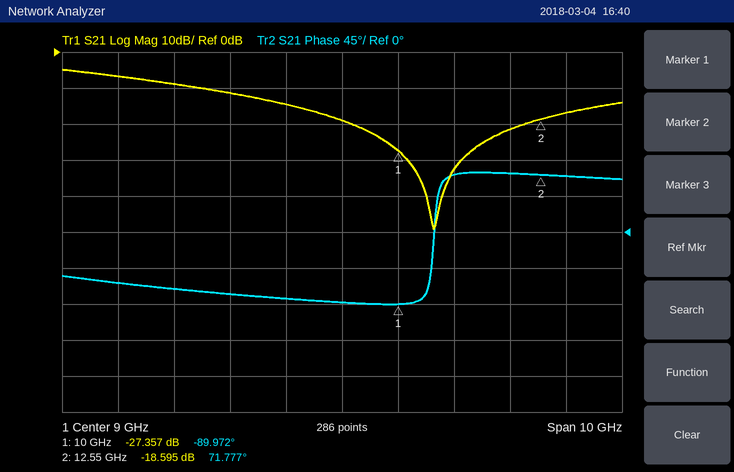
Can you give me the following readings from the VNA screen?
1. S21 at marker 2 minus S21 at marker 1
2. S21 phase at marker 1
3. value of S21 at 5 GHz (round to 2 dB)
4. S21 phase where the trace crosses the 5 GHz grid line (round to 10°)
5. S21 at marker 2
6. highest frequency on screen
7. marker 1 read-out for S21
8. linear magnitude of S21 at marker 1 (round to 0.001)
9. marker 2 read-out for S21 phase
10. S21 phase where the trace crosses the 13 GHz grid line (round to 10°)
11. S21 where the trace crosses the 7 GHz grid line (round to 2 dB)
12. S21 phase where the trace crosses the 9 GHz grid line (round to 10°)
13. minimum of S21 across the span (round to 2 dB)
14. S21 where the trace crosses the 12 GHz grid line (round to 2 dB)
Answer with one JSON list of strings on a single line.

["8.762 dB", "-89.972°", "-6 dB", "-60°", "-18.595 dB", "14 GHz", "-27.357 dB", "0.043", "71.777°", "70°", "-12 dB", "-90°", "-50 dB", "-22 dB"]
